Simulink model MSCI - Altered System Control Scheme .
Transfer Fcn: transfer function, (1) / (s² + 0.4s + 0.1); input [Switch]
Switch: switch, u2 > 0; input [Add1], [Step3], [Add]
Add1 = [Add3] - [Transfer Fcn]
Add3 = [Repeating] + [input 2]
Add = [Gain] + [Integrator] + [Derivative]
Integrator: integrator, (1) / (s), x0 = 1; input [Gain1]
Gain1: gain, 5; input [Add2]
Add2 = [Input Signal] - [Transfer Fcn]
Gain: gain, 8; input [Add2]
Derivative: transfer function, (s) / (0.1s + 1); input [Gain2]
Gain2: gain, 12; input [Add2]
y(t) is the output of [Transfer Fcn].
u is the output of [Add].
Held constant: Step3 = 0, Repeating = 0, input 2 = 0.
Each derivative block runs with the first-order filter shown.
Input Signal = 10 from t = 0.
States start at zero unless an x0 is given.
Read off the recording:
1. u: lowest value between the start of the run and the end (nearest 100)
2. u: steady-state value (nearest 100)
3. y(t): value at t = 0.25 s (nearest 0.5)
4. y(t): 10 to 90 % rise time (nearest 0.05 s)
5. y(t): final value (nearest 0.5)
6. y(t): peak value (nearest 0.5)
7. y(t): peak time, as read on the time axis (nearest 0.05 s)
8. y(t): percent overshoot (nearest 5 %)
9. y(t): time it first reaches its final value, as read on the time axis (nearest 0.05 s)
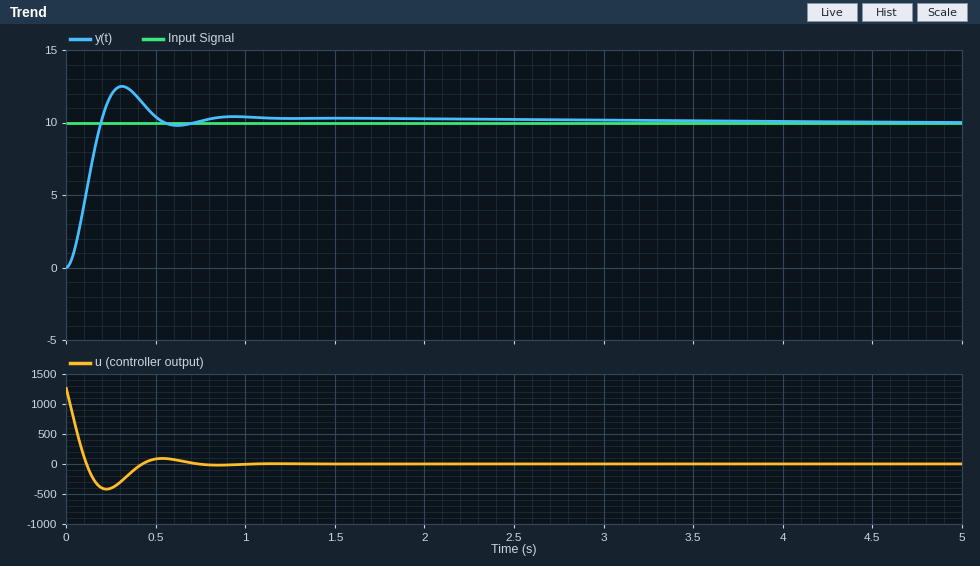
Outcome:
-400
0
12.0
0.15 s
10.0
12.5
0.30 s
25 %
0.20 s
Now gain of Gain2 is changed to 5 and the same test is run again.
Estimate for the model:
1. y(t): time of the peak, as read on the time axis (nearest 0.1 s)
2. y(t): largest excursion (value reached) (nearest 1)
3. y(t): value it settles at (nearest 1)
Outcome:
0.6 s
13
10
